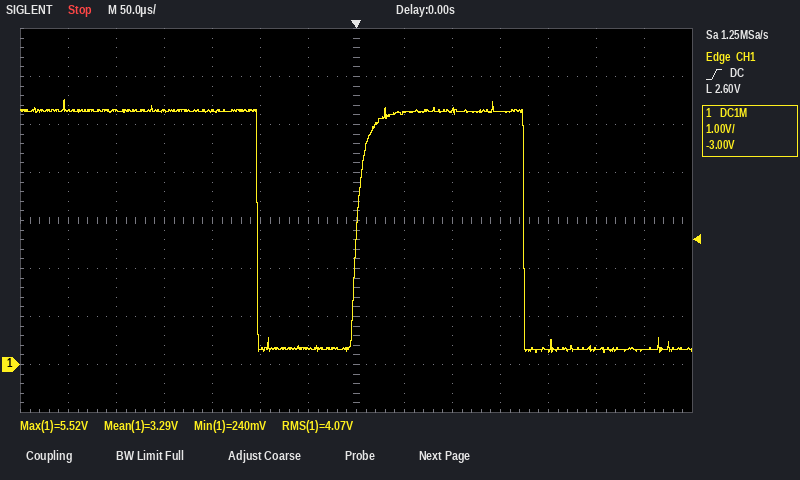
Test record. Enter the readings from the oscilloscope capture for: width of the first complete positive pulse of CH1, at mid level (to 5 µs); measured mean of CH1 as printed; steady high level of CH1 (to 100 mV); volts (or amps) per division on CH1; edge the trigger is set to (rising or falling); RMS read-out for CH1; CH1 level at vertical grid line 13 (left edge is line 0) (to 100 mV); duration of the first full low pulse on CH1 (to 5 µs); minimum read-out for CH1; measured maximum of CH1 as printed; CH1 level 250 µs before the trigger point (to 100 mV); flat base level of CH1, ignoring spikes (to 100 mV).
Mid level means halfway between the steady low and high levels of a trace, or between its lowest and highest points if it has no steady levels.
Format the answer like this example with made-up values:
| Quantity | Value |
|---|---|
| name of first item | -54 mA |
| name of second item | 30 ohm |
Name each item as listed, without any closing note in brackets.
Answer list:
| Quantity | Value |
|---|---|
| width of the first complete positive pulse of CH1, at mid level | 175 µs |
| measured mean of CH1 as printed | 3.29 V |
| steady high level of CH1 | 5.3 V |
| volts (or amps) per division on CH1 | 1 V |
| edge the trigger is set to | rising |
| RMS read-out for CH1 | 4.07 V |
| CH1 level at vertical grid line 13 (left edge is line 0) | 300 mV |
| duration of the first full low pulse on CH1 | 105 µs |
| minimum read-out for CH1 | 240 mV |
| measured maximum of CH1 as printed | 5.52 V |
| CH1 level 250 µs before the trigger point | 5.3 V |
| flat base level of CH1, ignoring spikes | 300 mV |
